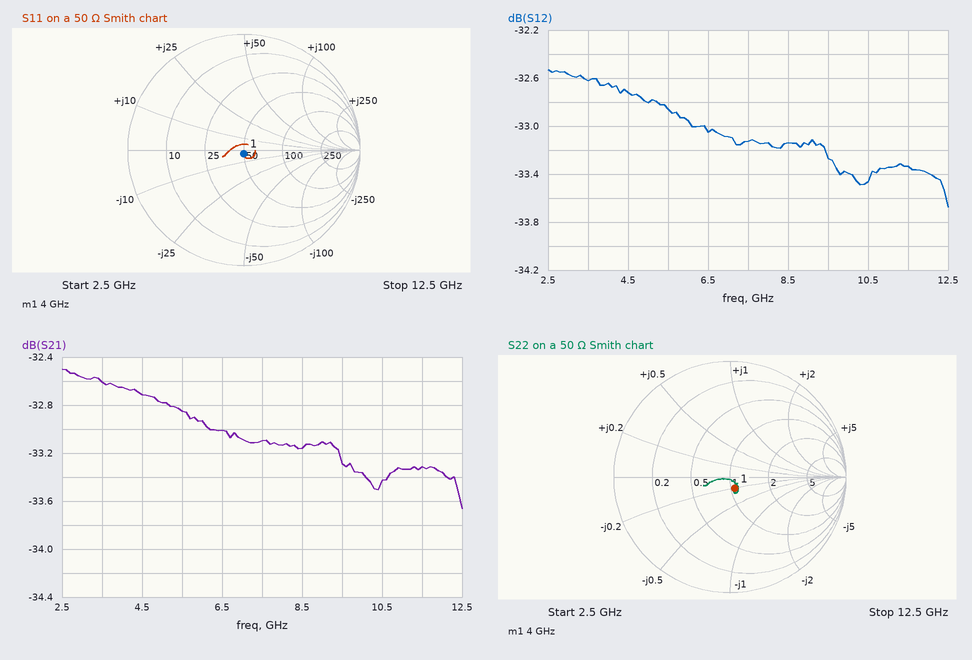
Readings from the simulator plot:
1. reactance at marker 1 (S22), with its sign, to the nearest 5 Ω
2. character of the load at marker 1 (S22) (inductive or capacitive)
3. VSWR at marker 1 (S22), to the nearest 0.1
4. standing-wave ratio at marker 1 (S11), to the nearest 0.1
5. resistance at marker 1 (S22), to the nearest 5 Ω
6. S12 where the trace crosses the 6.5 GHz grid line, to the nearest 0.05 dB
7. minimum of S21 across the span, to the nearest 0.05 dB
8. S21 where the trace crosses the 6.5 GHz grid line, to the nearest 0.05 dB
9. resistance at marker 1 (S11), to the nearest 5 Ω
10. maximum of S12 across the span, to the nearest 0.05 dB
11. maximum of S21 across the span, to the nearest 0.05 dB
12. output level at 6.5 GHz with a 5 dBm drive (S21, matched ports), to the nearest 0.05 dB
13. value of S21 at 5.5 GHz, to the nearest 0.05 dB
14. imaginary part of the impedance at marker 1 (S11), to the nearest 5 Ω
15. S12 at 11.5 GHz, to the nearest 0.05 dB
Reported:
-10 Ω
capacitive
1.2
1.1
55 Ω
-33.05 dB
-33.65 dB
-33.00 dB
50 Ω
-32.55 dB
-32.50 dB
-28.00 dBm
-32.85 dB
-5 Ω
-33.35 dB
